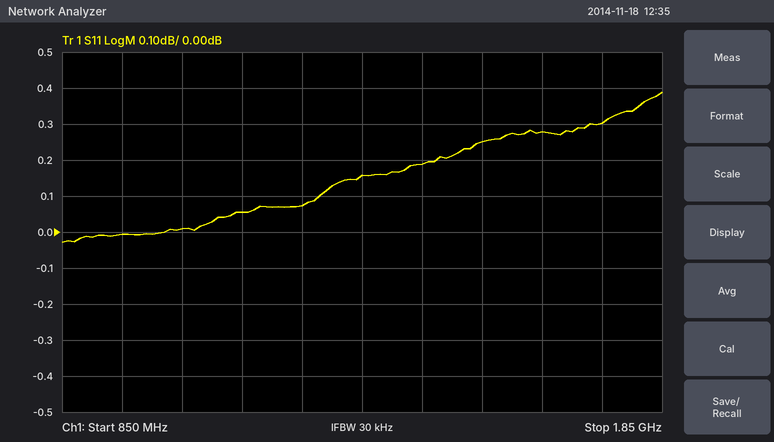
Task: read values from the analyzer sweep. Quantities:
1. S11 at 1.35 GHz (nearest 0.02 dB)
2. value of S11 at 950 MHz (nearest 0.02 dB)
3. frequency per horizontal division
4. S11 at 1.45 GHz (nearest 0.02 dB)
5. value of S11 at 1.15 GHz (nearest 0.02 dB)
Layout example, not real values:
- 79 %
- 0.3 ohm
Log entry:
- 0.16 dB
- 0.00 dB
- 100 MHz
- 0.18 dB
- 0.06 dB
